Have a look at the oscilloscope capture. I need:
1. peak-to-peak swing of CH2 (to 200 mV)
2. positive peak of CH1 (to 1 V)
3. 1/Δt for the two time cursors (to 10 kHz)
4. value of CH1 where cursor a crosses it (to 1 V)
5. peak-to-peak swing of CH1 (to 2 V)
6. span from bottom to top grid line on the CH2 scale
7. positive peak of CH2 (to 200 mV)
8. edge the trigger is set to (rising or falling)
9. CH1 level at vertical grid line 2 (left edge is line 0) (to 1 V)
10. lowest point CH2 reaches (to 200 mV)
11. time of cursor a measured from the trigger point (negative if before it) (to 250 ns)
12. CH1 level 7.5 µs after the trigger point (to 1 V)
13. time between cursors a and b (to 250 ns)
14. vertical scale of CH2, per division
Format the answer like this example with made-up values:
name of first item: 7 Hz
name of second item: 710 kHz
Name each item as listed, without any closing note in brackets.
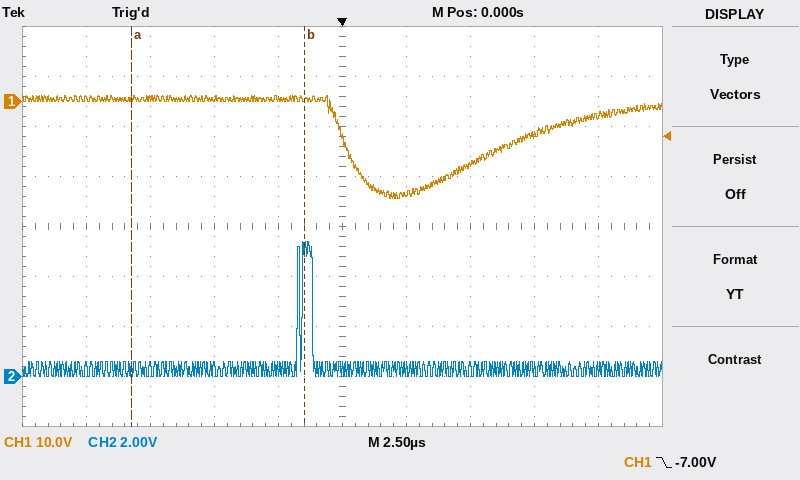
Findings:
peak-to-peak swing of CH2: 5.4 V
positive peak of CH1: 1 V
1/Δt for the two time cursors: 150 kHz
value of CH1 where cursor a crosses it: 1 V
peak-to-peak swing of CH1: 20 V
span from bottom to top grid line on the CH2 scale: 16 V
positive peak of CH2: 5.4 V
edge the trigger is set to: falling
CH1 level at vertical grid line 2 (left edge is line 0): 1 V
lowest point CH2 reaches: 0.0 V
time of cursor a measured from the trigger point (negative if before it): -8.25 µs
CH1 level 7.5 µs after the trigger point: -7 V
time between cursors a and b: 6.75 µs
vertical scale of CH2, per division: 2 V
